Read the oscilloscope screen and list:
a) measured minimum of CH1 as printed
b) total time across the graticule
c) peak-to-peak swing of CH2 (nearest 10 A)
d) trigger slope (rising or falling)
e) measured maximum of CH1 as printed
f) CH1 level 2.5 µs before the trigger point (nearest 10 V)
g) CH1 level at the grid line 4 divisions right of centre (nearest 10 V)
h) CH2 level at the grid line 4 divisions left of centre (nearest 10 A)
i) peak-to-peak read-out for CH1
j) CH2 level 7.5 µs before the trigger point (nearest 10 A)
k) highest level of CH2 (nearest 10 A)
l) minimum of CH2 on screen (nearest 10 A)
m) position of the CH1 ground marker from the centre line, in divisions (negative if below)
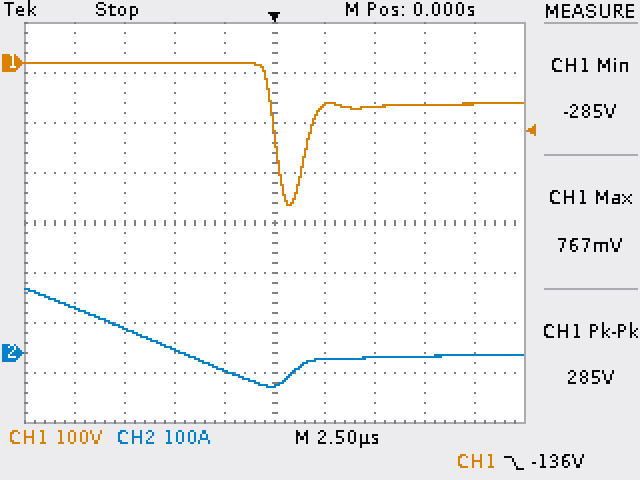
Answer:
-285 V
25 µs
200 A
falling
767 mV
0 V
-80 V
90 A
285 V
50 A
130 A
-70 A
+3.2 div
